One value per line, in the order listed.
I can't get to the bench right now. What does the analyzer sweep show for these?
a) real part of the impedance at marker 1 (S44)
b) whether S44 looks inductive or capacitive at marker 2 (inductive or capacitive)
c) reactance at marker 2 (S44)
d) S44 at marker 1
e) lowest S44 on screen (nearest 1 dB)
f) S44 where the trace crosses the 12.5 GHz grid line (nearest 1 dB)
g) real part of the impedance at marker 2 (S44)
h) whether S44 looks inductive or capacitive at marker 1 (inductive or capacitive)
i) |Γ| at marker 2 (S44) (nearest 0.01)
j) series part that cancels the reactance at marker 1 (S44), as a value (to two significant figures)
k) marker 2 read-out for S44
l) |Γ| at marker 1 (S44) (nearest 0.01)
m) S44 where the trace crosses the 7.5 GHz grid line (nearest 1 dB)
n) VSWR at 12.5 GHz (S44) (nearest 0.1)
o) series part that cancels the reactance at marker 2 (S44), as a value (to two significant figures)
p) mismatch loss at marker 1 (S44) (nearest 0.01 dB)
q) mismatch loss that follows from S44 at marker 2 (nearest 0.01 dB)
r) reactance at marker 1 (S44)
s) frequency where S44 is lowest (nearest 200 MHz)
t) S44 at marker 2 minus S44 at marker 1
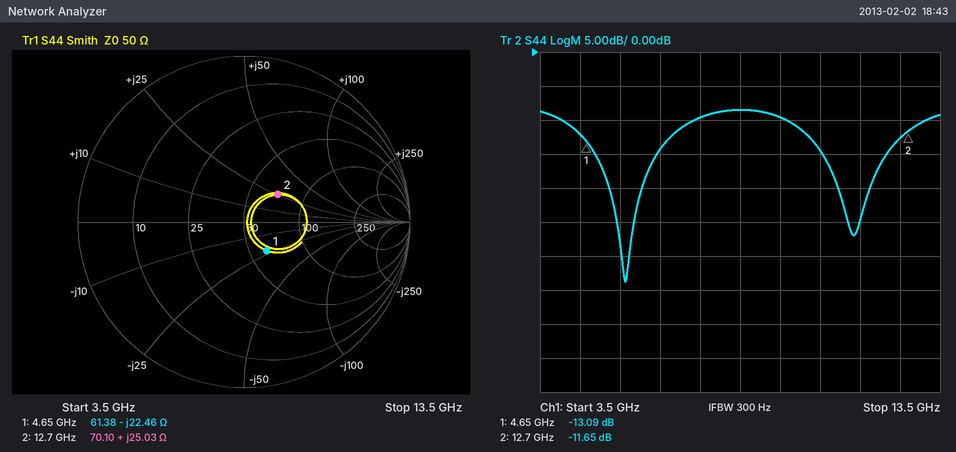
61.38 Ω
inductive
+25.03 Ω
-13.09 dB
-34 dB
-13 dB
70.10 Ω
capacitive
0.26
770 pH
-11.65 dB
0.22
-10 dB
1.6
500 fF
0.22 dB
0.31 dB
-22.46 Ω
5.6 GHz
1.44 dB
